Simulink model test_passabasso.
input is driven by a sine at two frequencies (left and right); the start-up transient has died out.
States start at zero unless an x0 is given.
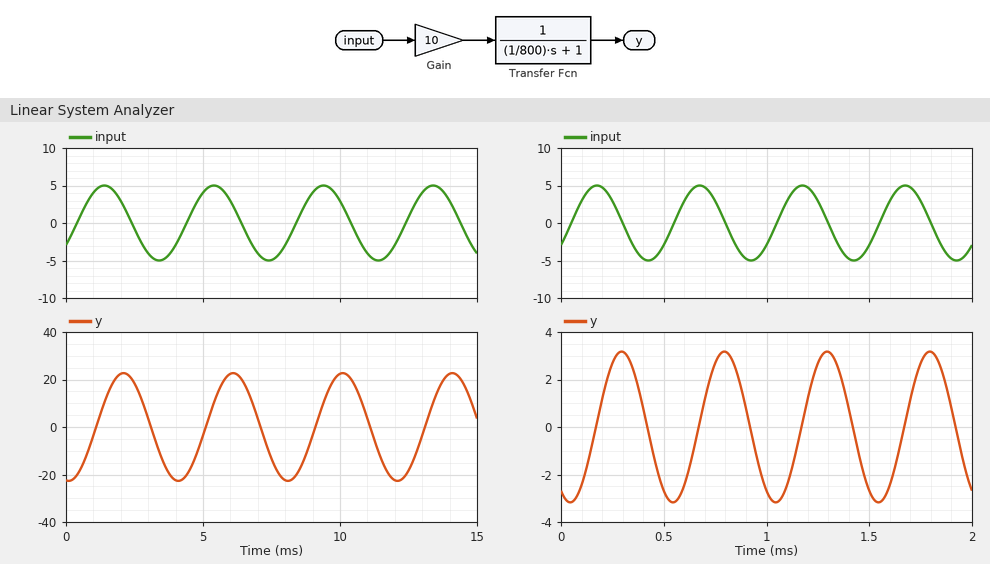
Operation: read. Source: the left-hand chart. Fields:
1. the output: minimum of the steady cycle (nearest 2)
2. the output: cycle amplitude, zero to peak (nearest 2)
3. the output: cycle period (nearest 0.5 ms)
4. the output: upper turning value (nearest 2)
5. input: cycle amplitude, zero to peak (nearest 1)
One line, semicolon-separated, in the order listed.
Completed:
-22; 22; 4.0 ms; 22; 5
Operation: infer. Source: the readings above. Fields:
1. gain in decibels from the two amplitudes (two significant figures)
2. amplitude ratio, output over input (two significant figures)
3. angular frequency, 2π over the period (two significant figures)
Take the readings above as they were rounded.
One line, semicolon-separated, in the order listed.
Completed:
13 dB; 4.4; 1.6 rad/ms
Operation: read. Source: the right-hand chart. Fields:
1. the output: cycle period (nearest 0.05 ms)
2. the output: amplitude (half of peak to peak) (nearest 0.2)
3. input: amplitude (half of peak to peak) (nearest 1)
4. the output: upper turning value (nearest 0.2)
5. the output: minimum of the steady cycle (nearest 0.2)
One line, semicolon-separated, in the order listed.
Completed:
0.50 ms; 3.2; 5; 3.2; -3.2
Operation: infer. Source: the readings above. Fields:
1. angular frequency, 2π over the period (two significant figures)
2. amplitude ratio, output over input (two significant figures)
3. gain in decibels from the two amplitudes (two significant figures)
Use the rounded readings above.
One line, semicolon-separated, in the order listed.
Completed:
13 rad/ms; 0.64; -3.9 dB
